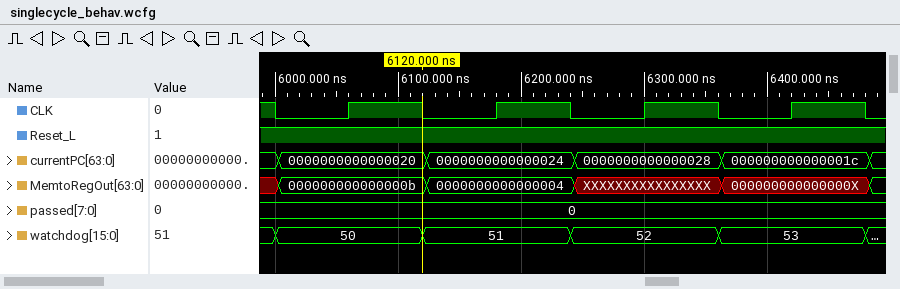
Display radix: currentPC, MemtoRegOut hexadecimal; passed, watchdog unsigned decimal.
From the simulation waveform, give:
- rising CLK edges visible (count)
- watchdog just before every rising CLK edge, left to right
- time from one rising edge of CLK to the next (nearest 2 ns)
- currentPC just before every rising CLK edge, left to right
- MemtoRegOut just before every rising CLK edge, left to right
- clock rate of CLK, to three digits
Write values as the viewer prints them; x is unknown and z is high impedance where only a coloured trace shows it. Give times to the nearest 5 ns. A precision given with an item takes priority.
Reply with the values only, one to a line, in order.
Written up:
4
50, 51, 52, 53
120 ns
0000000000000020, 0000000000000024, 0000000000000028, 000000000000001c
000000000000000b, 0000000000000004, XXXXXXXXXXXXXXXX, 000000000000000X
8.33 MHz
